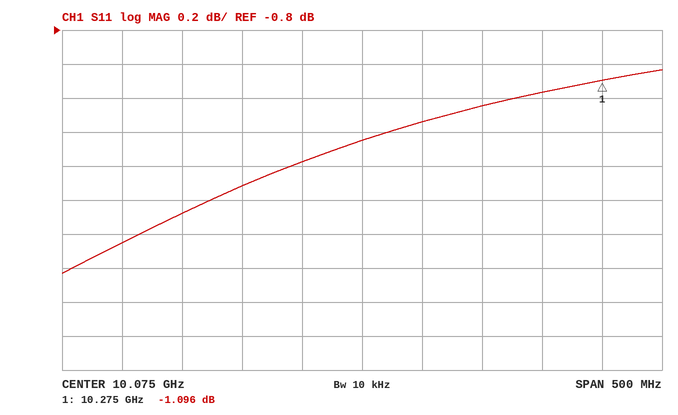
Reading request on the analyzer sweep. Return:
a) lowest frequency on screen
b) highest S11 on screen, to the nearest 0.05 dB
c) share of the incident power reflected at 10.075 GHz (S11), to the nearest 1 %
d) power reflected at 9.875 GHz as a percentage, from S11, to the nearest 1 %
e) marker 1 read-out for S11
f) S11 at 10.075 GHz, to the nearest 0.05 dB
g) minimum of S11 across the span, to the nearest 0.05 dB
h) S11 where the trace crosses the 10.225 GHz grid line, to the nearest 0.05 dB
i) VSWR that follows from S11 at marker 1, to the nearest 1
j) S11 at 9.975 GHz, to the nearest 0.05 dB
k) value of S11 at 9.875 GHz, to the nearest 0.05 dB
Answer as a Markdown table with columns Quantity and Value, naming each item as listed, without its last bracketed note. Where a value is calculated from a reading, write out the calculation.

| Quantity | Value |
|---|---|
| lowest frequency on screen | 9.825 GHz |
| highest S11 on screen, to the nearest 0.05 dB | -1.05 dB |
| share of the incident power reflected at 10.075 GHz (S11), to the nearest 1 % | 10^(-1.45/10) ≈ 72 % |
| power reflected at 9.875 GHz as a percentage, from S11, to the nearest 1 % | 10^(-2.05/10) ≈ 62 % |
| marker 1 read-out for S11 | -1.096 dB |
| S11 at 10.075 GHz, to the nearest 0.05 dB | -1.45 dB |
| minimum of S11 across the span, to the nearest 0.05 dB | -2.25 dB |
| S11 where the trace crosses the 10.225 GHz grid line, to the nearest 0.05 dB | -1.15 dB |
| VSWR that follows from S11 at marker 1, to the nearest 1 | (1 + 0.8815)/(1 − 0.8815) ≈ 16 |
| S11 at 9.975 GHz, to the nearest 0.05 dB | -1.70 dB |
| value of S11 at 9.875 GHz, to the nearest 0.05 dB | -2.05 dB |
